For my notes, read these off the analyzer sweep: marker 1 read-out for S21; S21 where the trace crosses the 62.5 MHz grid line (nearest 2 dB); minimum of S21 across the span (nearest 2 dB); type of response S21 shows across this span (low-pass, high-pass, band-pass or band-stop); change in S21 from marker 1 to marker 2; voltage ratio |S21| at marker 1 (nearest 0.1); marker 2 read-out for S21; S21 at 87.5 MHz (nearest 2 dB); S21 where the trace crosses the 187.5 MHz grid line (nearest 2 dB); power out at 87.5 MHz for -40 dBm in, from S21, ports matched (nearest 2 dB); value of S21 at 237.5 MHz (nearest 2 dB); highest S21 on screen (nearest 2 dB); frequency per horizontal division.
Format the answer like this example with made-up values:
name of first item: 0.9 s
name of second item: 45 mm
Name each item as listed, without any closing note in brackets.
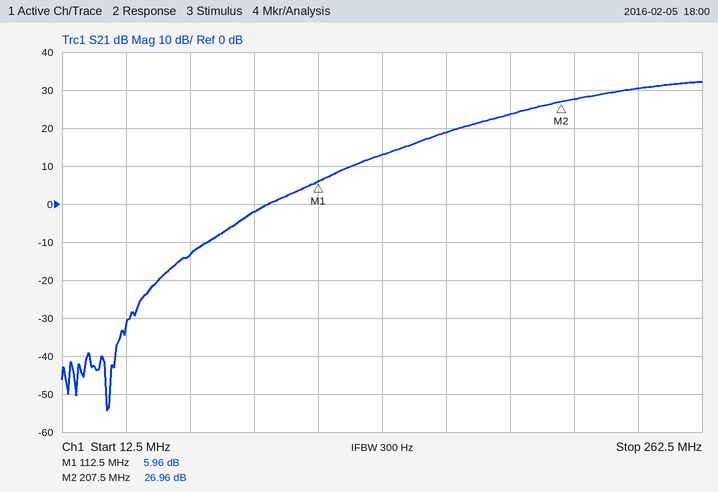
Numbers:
marker 1 read-out for S21: 5.96 dB
S21 where the trace crosses the 62.5 MHz grid line: -14 dB
minimum of S21 across the span: -54 dB
type of response S21 shows across this span: high-pass
change in S21 from marker 1 to marker 2: 21.00 dB
voltage ratio |S21| at marker 1: 2.0
marker 2 read-out for S21: 26.96 dB
S21 at 87.5 MHz: -2 dB
S21 where the trace crosses the 187.5 MHz grid line: 24 dB
power out at 87.5 MHz for -40 dBm in, from S21, ports matched: -42 dBm
value of S21 at 237.5 MHz: 30 dB
highest S21 on screen: 32 dB
frequency per horizontal division: 25 MHz
